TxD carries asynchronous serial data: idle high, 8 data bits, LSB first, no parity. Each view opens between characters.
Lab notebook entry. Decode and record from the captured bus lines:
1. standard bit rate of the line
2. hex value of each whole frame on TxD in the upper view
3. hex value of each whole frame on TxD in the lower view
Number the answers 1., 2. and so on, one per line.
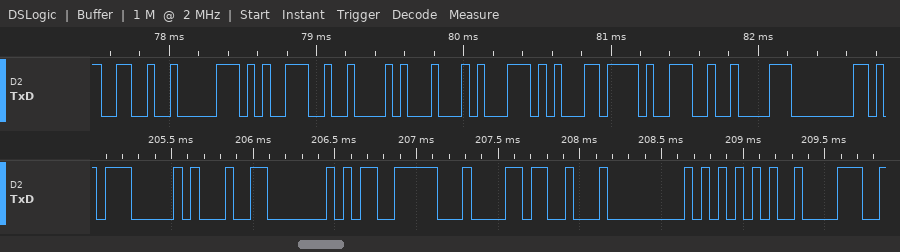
1. 19200 baud
2. 26, 70, 39, 42, 44, 5C, EC, 39, C2, 80
3. 07, 91, 40, F3, 84, 13, 00, 55, C2
